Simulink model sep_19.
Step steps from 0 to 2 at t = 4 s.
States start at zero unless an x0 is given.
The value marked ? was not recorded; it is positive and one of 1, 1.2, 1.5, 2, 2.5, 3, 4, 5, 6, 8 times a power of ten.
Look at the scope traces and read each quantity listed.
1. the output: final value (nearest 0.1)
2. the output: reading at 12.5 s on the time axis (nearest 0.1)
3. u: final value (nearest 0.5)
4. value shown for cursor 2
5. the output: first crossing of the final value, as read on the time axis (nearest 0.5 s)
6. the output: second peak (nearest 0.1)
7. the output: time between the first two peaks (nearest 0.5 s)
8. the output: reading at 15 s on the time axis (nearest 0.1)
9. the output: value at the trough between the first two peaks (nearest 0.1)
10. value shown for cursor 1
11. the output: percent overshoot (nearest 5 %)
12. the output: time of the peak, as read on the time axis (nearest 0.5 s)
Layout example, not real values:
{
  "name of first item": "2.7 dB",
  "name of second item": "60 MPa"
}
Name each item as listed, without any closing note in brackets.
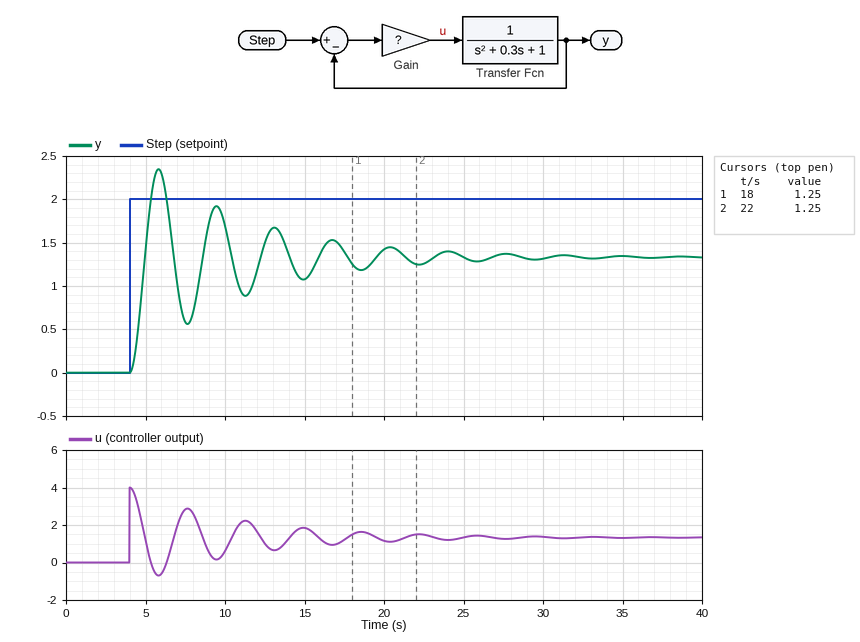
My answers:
{
  "the output: final value": "1.3",
  "the output: reading at 12.5 s on the time axis": "1.5",
  "u: final value": "1.5",
  "value shown for cursor 2": "1.25",
  "the output: first crossing of the final value, as read on the time axis": "5.0 s",
  "the output: second peak": "1.9",
  "the output: time between the first two peaks": "3.5 s",
  "the output: reading at 15 s on the time axis": "1.1",
  "the output: value at the trough between the first two peaks": "0.6",
  "value shown for cursor 1": "1.25",
  "the output: percent overshoot": "75 %",
  "the output: time of the peak, as read on the time axis": "6.0 s"
}
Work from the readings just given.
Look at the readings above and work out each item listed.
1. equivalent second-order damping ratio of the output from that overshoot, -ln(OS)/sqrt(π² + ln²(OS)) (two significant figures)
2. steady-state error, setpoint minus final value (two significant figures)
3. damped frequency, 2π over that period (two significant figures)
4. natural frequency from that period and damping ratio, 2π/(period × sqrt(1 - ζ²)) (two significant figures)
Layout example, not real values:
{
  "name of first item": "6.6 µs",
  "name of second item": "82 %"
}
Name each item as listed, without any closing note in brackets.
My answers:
{
  "equivalent second-order damping ratio of the output from that overshoot, -ln(OS)/sqrt(π² + ln²(OS))": "0.091",
  "steady-state error, setpoint minus final value": "0.70",
  "damped frequency, 2π over that period": "1.8 rad/s",
  "natural frequency from that period and damping ratio, 2π/(period × sqrt(1 - ζ²))": "1.8 rad/s"
}
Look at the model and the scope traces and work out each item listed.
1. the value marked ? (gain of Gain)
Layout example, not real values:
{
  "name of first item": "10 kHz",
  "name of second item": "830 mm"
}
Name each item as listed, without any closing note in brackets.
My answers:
{
  "the value marked ?": "2"
}
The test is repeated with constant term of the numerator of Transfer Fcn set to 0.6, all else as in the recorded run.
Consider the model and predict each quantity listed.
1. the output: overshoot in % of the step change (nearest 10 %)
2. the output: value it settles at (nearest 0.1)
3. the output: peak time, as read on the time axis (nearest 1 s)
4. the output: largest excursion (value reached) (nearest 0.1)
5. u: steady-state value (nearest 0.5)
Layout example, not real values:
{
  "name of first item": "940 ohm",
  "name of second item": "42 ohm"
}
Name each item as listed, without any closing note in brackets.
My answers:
{
  "the output: overshoot in % of the step change": "70 %",
  "the output: value it settles at": "1.1",
  "the output: peak time, as read on the time axis": "6 s",
  "the output: largest excursion (value reached)": "1.9",
  "u: steady-state value": "2.0"
}
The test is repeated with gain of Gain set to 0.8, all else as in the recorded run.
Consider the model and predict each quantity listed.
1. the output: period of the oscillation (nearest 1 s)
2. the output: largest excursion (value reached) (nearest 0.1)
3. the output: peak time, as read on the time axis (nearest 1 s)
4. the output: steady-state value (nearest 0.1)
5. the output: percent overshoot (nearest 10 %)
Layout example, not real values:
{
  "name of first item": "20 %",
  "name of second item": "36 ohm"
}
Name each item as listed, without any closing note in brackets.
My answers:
{
  "the output: period of the oscillation": "5 s",
  "the output: largest excursion (value reached)": "1.5",
  "the output: peak time, as read on the time axis": "6 s",
  "the output: steady-state value": "0.9",
  "the output: percent overshoot": "70 %"
}
